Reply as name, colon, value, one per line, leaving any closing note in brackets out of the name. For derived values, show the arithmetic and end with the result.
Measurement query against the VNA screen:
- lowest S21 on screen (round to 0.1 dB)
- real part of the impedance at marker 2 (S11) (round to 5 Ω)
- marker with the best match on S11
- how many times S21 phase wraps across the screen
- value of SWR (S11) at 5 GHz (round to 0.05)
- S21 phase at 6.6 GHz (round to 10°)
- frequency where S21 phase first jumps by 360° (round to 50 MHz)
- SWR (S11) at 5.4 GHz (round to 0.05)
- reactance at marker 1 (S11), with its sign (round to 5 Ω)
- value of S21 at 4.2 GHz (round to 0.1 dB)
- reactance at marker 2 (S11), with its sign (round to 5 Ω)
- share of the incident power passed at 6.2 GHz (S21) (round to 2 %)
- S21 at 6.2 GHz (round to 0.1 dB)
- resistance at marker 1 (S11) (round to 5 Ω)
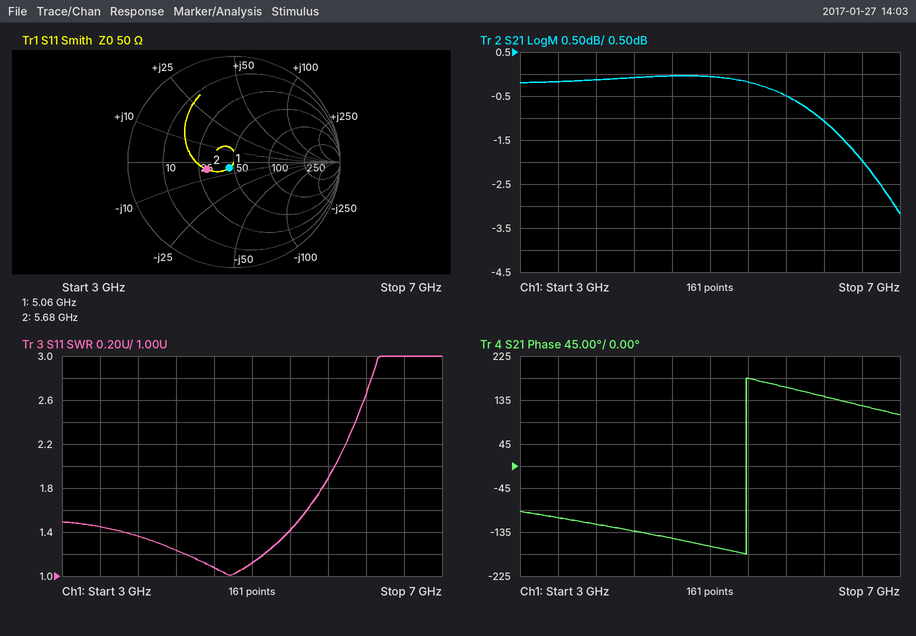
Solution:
lowest S21 on screen: -3.2 dB
real part of the impedance at marker 2 (S11): 30 Ω
marker with the best match on S11: marker 1
how many times S21 phase wraps across the screen: 1
value of SWR (S11) at 5 GHz: 1.10
S21 phase at 6.6 GHz: 120°
frequency where S21 phase first jumps by 360°: 5.40 GHz
SWR (S11) at 5.4 GHz: 1.40
reactance at marker 1 (S11), with its sign: -5 Ω
value of S21 at 4.2 GHz: -0.1 dB
reactance at marker 2 (S11), with its sign: -5 Ω
share of the incident power passed at 6.2 GHz (S21): 10^(-1.1/10) ≈ 78 %
S21 at 6.2 GHz: -1.1 dB
resistance at marker 1 (S11): 45 Ω
